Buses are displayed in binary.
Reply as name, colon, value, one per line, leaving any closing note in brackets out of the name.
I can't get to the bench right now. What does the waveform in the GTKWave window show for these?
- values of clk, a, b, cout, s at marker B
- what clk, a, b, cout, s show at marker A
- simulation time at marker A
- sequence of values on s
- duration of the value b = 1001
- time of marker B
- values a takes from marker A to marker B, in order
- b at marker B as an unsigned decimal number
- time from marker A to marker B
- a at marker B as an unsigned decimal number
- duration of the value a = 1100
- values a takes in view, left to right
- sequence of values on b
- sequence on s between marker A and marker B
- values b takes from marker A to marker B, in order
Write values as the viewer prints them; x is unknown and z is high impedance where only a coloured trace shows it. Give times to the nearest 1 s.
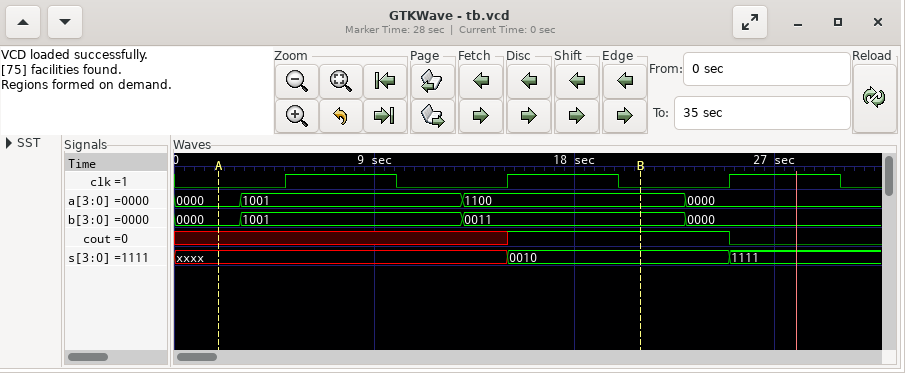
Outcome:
values of clk, a, b, cout, s at marker B: clk=0, a=1100, b=0011, cout=1, s=0010
what clk, a, b, cout, s show at marker A: clk=0, a=0000, b=0000, cout=x, s=xxxx
simulation time at marker A: 2 s
sequence of values on s: xxxx, 0010, 1111
duration of the value b = 1001: 10 s
time of marker B: 21 s
values a takes from marker A to marker B, in order: 0000, 1001, 1100
b at marker B as an unsigned decimal number: 3
time from marker A to marker B: 19 s
a at marker B as an unsigned decimal number: 12
duration of the value a = 1100: 10 s
values a takes in view, left to right: 0000, 1001, 1100, 0000
sequence of values on b: 0000, 1001, 0011, 0000
sequence on s between marker A and marker B: xxxx, 0010
values b takes from marker A to marker B, in order: 0000, 1001, 0011
